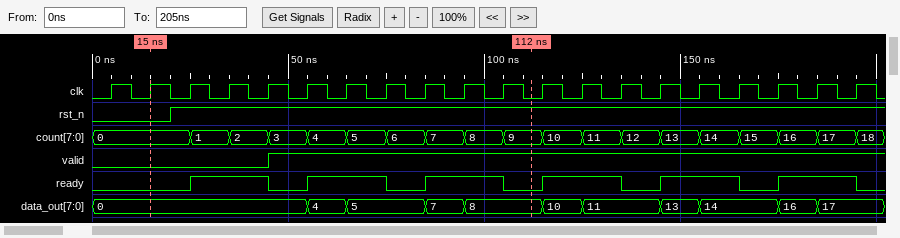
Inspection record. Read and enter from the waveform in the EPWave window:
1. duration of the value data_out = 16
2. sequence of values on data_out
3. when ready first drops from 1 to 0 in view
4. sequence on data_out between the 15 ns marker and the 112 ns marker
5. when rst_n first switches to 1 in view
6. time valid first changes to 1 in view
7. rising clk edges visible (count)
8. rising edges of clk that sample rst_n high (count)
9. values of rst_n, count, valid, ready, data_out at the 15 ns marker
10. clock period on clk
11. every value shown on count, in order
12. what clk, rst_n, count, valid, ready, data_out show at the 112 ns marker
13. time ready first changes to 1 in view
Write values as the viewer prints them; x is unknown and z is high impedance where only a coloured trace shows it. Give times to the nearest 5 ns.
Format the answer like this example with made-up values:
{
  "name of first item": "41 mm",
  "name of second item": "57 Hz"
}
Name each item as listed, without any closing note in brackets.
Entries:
{
  "duration of the value data_out = 16": "10 ns",
  "sequence of values on data_out": "0, 4, 5, 7, 8, 10, 11, 13, 14, 16, 17",
  "when ready first drops from 1 to 0 in view": "45 ns",
  "sequence on data_out between the 15 ns marker and the 112 ns marker": "0, 4, 5, 7, 8",
  "when rst_n first switches to 1 in view": "20 ns",
  "time valid first changes to 1 in view": "45 ns",
  "rising clk edges visible": "20",
  "rising edges of clk that sample rst_n high": "18",
  "values of rst_n, count, valid, ready, data_out at the 15 ns marker": "rst_n=0, count=0, valid=0, ready=0, data_out=0",
  "clock period on clk": "10 ns",
  "every value shown on count, in order": "0, 1, 2, 3, 4, 5, 6, 7, 8, 9, 10, 11, 12, 13, 14, 15, 16, 17, 18",
  "what clk, rst_n, count, valid, ready, data_out show at the 112 ns marker": "clk=0, rst_n=1, count=9, valid=1, ready=0, data_out=8",
  "time ready first changes to 1 in view": "25 ns"
}
